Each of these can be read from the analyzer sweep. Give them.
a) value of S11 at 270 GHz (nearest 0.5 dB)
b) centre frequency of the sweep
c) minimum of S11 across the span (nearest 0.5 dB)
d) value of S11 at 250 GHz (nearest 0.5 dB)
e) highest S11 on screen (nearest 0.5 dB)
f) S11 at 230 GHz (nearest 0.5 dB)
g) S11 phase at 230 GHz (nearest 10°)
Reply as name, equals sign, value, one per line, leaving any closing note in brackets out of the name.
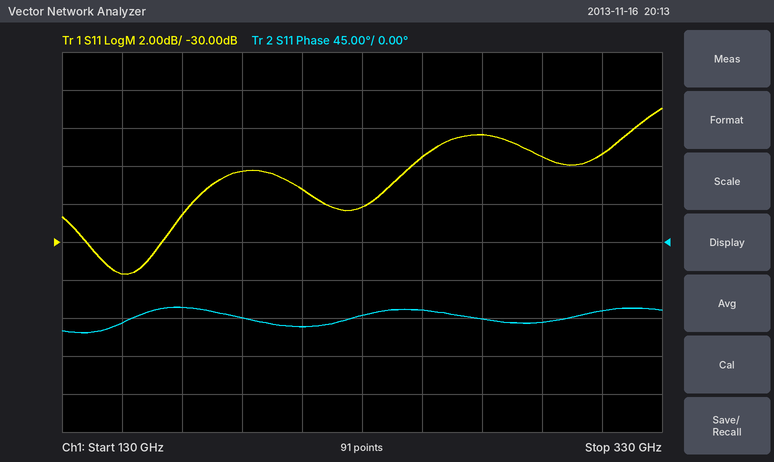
value of S11 at 270 GHz = -24.5 dB
centre frequency of the sweep = 230 GHz
minimum of S11 across the span = -31.5 dB
value of S11 at 250 GHz = -25.5 dB
highest S11 on screen = -23.0 dB
S11 at 230 GHz = -28.0 dB
S11 phase at 230 GHz = -90°
